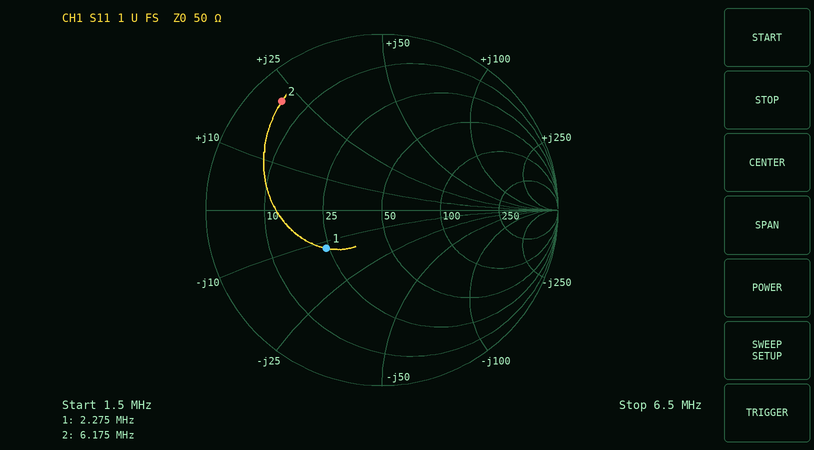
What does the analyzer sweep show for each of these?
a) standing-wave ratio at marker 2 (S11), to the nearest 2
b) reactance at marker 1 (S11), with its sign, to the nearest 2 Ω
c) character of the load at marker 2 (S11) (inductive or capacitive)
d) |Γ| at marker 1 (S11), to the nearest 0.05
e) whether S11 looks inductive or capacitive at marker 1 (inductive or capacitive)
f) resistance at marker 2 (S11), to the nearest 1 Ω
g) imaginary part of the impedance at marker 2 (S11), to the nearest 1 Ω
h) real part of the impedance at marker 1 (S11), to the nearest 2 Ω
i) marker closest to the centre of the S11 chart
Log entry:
12
-12 Ω
inductive
0.40
capacitive
5 Ω
+22 Ω
24 Ω
marker 1
